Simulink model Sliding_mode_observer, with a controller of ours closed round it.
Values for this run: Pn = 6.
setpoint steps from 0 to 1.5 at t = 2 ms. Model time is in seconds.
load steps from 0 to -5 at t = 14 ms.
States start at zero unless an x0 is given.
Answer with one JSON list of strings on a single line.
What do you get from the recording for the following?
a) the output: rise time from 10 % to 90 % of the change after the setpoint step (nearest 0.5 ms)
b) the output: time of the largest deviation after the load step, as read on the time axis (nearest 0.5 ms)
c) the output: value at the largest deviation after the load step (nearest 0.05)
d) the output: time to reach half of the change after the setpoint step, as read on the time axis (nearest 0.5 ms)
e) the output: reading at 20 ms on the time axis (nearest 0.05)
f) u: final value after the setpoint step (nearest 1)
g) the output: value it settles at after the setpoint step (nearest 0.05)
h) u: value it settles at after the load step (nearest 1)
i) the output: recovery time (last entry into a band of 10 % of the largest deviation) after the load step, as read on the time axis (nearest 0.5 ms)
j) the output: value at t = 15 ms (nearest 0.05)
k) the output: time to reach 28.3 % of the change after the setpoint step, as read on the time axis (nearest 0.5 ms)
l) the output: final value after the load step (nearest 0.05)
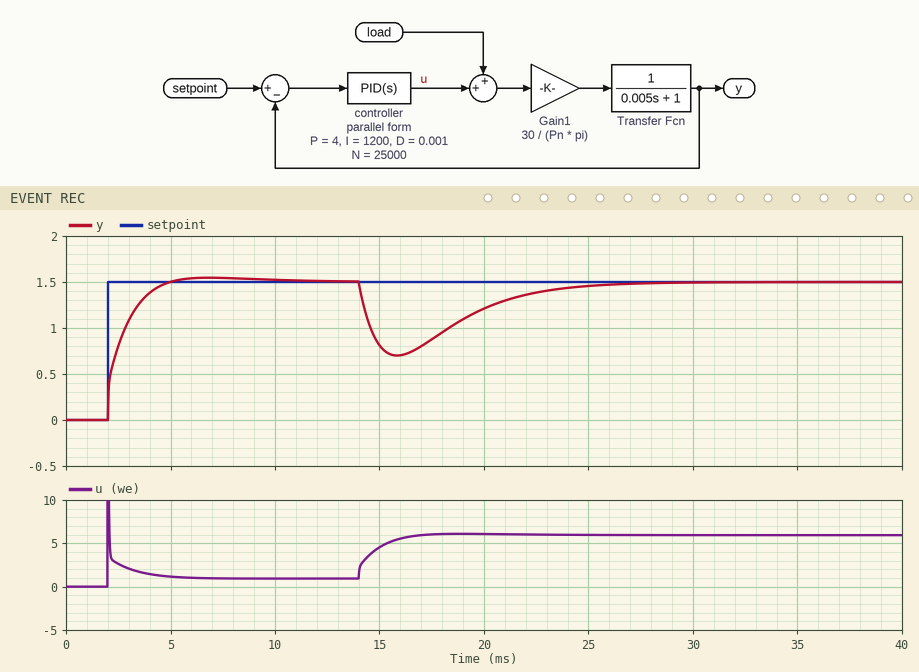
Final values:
["2.0 ms", "16.0 ms", "0.70", "2.5 ms", "1.20", "1", "1.50", "6", "23.5 ms", "0.80", "2.0 ms", "1.50"]
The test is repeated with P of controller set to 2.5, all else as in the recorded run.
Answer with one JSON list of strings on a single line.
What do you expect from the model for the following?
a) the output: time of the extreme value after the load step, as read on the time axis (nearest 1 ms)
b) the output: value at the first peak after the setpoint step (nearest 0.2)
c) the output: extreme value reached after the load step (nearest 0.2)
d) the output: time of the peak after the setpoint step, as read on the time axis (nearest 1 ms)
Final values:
["16 ms", "1.6", "0.4", "7 ms"]
